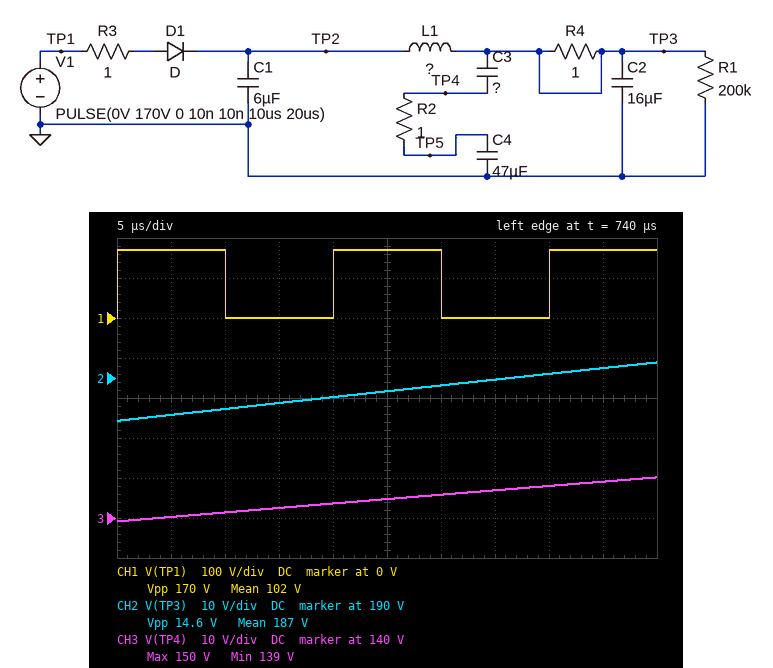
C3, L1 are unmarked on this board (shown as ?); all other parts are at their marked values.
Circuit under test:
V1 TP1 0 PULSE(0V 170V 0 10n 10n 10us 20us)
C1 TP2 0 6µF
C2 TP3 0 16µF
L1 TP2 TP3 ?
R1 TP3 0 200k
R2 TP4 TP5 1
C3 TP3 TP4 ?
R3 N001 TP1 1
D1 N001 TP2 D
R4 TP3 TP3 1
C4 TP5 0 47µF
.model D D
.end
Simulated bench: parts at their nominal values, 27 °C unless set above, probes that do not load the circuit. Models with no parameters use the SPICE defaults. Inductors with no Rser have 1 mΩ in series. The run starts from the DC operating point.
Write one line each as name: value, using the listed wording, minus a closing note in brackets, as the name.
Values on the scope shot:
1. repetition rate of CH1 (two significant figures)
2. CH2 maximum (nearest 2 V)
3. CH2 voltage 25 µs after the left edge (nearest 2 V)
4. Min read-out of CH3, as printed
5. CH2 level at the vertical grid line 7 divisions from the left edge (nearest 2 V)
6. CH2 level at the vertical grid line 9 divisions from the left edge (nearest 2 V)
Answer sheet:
repetition rate of CH1: 50 kHz
CH2 maximum: 194 V
CH2 voltage 25 µs after the left edge: 186 V
Min read-out of CH3, as printed: 139 V
CH2 level at the vertical grid line 7 divisions from the left edge: 190 V
CH2 level at the vertical grid line 9 divisions from the left edge: 192 V
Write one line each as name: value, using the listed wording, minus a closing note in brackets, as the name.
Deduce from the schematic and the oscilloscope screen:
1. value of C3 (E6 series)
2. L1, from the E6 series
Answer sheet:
value of C3: 150 µF
L1, from the E6 series: 3.3 mH
